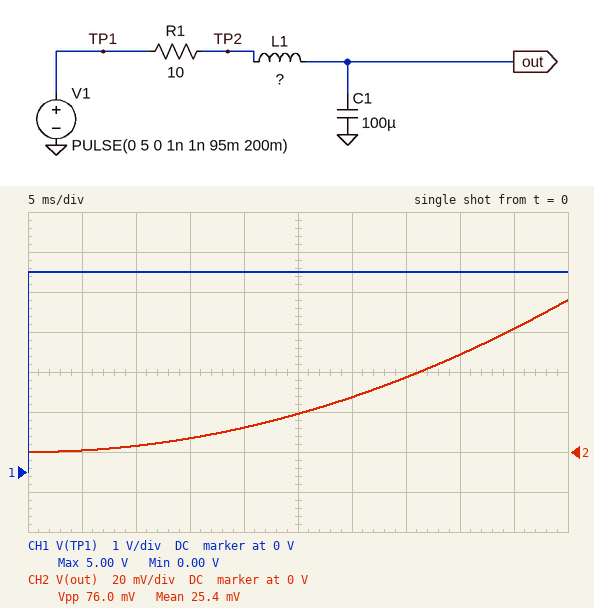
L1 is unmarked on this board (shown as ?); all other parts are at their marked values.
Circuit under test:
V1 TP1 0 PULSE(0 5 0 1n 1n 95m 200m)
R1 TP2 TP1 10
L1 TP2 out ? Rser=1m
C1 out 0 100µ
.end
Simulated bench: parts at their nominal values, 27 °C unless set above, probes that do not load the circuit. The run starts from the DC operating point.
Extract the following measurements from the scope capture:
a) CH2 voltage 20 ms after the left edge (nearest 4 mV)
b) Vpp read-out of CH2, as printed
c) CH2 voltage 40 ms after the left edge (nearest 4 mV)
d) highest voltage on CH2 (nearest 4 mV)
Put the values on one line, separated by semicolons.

12 mV; 76.0 mV; 48 mV; 76 mV
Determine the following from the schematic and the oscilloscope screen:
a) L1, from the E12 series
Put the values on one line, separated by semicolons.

820 H
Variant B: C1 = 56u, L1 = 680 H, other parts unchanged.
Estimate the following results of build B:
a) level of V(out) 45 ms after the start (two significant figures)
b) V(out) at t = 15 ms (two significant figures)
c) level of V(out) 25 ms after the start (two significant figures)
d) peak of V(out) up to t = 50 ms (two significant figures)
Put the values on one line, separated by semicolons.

130 mV; 15 mV; 41 mV; 160 mV
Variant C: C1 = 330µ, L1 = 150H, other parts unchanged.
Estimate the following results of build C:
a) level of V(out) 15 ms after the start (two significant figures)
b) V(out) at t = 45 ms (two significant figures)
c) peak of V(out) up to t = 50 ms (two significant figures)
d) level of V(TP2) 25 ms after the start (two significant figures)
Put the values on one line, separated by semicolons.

11 mV; 100 mV; 130 mV; 5.0 V
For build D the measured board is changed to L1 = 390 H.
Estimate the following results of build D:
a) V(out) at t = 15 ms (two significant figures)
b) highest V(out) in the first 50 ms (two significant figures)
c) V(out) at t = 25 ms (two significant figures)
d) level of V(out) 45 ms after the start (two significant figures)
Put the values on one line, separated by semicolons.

14 mV; 160 mV; 40 mV; 130 mV
